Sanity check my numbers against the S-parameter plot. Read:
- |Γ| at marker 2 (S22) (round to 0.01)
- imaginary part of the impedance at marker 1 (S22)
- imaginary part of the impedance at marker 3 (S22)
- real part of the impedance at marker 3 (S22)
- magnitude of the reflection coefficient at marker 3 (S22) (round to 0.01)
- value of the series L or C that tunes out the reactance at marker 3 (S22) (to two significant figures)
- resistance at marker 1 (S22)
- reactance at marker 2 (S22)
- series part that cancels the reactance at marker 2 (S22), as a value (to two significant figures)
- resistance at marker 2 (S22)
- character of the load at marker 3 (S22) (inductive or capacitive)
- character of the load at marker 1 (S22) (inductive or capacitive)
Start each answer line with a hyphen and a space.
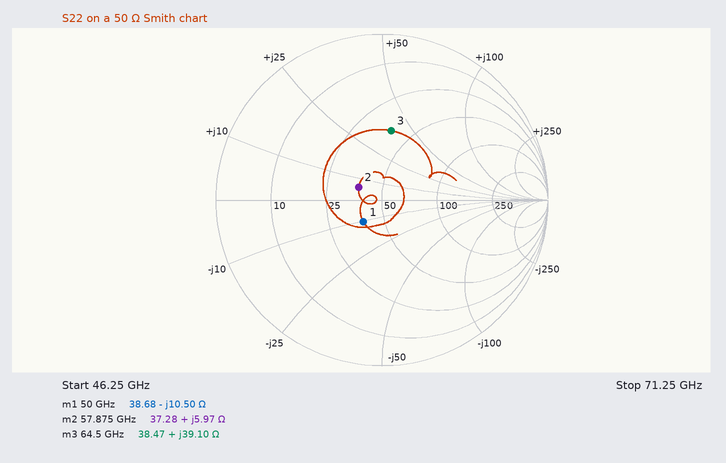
- 0.16
- -10.50 Ω
- +39.10 Ω
- 38.47 Ω
- 0.42
- 63 fF
- 38.68 Ω
- +5.97 Ω
- 460 fF
- 37.28 Ω
- inductive
- capacitive
